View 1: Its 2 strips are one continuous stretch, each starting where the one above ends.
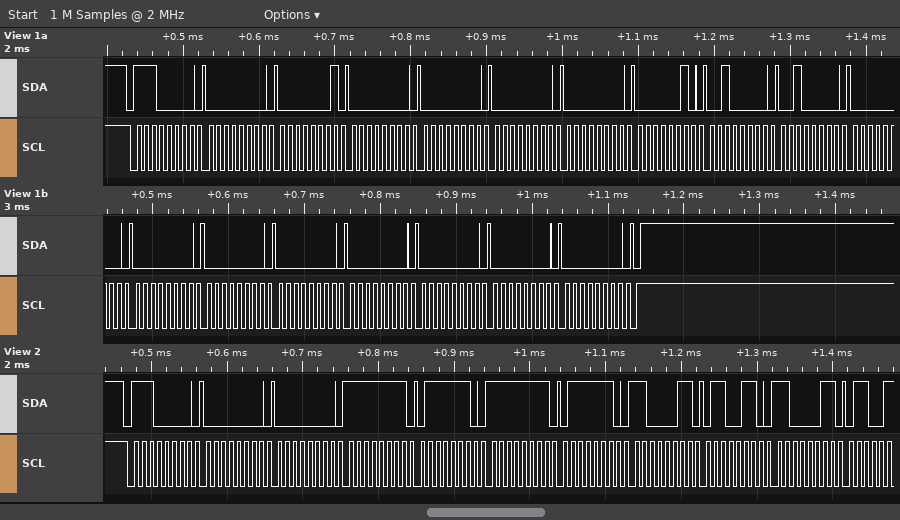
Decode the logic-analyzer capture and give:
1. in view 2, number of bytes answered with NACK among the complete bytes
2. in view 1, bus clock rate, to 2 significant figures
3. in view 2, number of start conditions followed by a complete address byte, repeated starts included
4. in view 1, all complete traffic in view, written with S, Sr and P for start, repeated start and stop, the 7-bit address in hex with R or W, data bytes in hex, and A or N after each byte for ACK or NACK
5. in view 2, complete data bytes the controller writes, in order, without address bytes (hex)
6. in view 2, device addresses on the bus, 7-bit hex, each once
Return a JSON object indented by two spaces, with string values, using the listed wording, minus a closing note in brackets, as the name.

{
  "in view 2, number of bytes answered with NACK among the complete bytes": "0",
  "in view 1, bus clock rate, to 2 significant figures": "100 kHz",
  "in view 2, number of start conditions followed by a complete address byte, repeated starts included": "1",
  "in view 1, all complete traffic in view, written with S, Sr and P for start, repeated start and stop, the 7-bit address in hex with R or W, data bytes in hex, and A or N after each byte for ACK or NACK": "S 70W A 00 A 01 A 00 A 00 A 00 A 00 A 02 A 20 A 20 A 00 A 00 A 00 A 00 A 00 A 00 A 00 A 00 A P",
  "in view 2, complete data bytes the controller writes, in order, without address bytes": "00 00 FF 7E FF 7E C3 66 C3",
  "in view 2, device addresses on the bus, 7-bit hex, each once": "0x70"
}
